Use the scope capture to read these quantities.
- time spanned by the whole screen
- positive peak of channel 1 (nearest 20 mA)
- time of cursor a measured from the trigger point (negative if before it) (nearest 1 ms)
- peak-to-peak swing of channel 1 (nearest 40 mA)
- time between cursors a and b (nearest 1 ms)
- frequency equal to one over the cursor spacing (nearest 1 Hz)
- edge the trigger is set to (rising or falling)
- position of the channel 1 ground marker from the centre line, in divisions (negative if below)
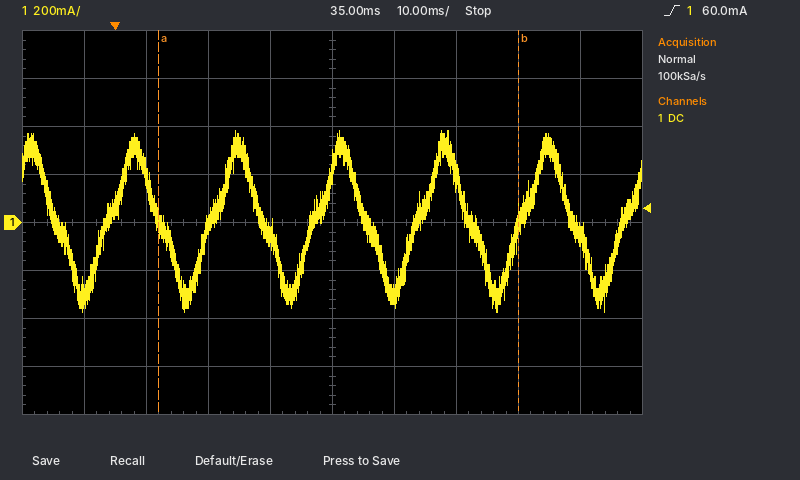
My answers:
100 ms
380 mA
+7 ms
760 mA
58 ms
17 Hz
rising
0.0 div
